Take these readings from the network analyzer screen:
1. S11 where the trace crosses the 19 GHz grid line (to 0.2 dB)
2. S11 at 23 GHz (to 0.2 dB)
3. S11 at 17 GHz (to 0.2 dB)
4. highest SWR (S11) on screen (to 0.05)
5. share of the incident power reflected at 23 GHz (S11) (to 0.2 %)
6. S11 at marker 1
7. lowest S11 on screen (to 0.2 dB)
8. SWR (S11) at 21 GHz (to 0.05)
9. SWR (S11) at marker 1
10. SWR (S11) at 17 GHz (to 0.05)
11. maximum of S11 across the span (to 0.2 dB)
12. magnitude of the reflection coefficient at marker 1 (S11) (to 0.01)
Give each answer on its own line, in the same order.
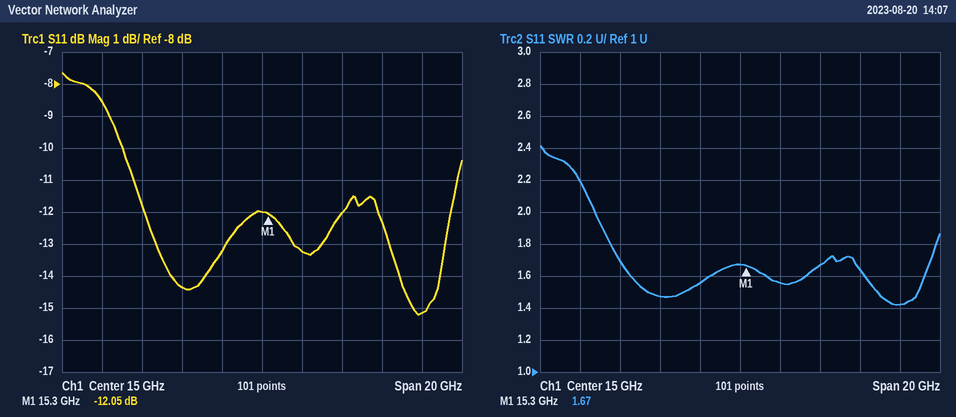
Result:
-12.0 dB
-15.2 dB
-13.2 dB
2.40
3.0 %
-12.05 dB
-15.2 dB
1.65
1.67
1.55
-7.6 dB
0.25
